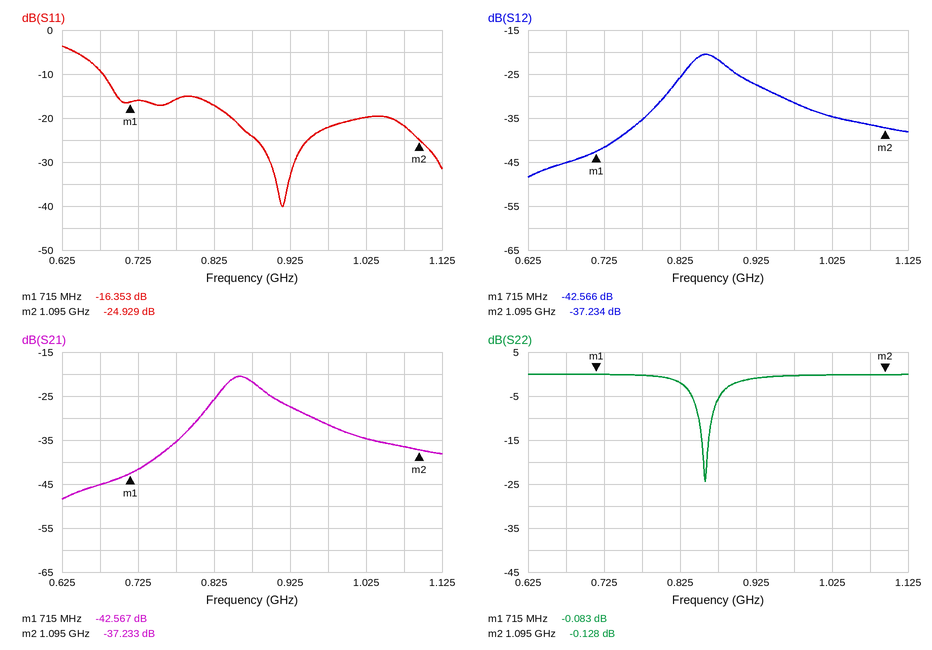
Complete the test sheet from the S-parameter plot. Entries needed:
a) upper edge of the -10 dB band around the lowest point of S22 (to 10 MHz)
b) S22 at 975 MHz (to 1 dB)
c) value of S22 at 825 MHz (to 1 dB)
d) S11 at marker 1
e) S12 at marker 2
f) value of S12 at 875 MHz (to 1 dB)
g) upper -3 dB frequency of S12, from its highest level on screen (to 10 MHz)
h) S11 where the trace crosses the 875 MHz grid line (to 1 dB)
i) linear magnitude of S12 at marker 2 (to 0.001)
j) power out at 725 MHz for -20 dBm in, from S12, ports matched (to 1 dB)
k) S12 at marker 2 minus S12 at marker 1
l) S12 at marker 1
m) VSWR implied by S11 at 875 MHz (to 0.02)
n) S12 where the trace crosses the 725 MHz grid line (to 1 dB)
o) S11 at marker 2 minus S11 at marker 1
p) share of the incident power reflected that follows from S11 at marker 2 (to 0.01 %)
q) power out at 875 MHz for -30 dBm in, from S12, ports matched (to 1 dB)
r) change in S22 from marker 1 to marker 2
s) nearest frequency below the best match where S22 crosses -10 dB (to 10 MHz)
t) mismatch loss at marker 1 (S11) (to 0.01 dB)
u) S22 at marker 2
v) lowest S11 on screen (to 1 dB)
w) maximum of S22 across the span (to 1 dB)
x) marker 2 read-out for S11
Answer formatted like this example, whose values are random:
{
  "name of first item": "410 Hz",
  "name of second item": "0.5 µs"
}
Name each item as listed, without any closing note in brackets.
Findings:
{
  "upper edge of the -10 dB band around the lowest point of S22": "870 MHz",
  "S22 at 975 MHz": "0 dB",
  "value of S22 at 825 MHz": "-2 dB",
  "S11 at marker 1": "-16.353 dB",
  "S12 at marker 2": "-37.234 dB",
  "value of S12 at 875 MHz": "-22 dB",
  "upper -3 dB frequency of S12, from its highest level on screen": "890 MHz",
  "S11 where the trace crosses the 875 MHz grid line": "-24 dB",
  "linear magnitude of S12 at marker 2": "0.014",
  "power out at 725 MHz for -20 dBm in, from S12, ports matched": "-62 dBm",
  "S12 at marker 2 minus S12 at marker 1": "5.332 dB",
  "S12 at marker 1": "-42.566 dB",
  "VSWR implied by S11 at 875 MHz": "1.14",
  "S12 where the trace crosses the 725 MHz grid line": "-42 dB",
  "S11 at marker 2 minus S11 at marker 1": "-8.576 dB",
  "share of the incident power reflected that follows from S11 at marker 2": "0.32 %",
  "power out at 875 MHz for -30 dBm in, from S12, ports matched": "-52 dBm",
  "change in S22 from marker 1 to marker 2": "-0.045 dB",
  "nearest frequency below the best match where S22 crosses -10 dB": "850 MHz",
  "mismatch loss at marker 1 (S11)": "0.10 dB",
  "S22 at marker 2": "-0.128 dB",
  "lowest S11 on screen": "-40 dB",
  "maximum of S22 across the span": "0 dB",
  "marker 2 read-out for S11": "-24.929 dB"
}
